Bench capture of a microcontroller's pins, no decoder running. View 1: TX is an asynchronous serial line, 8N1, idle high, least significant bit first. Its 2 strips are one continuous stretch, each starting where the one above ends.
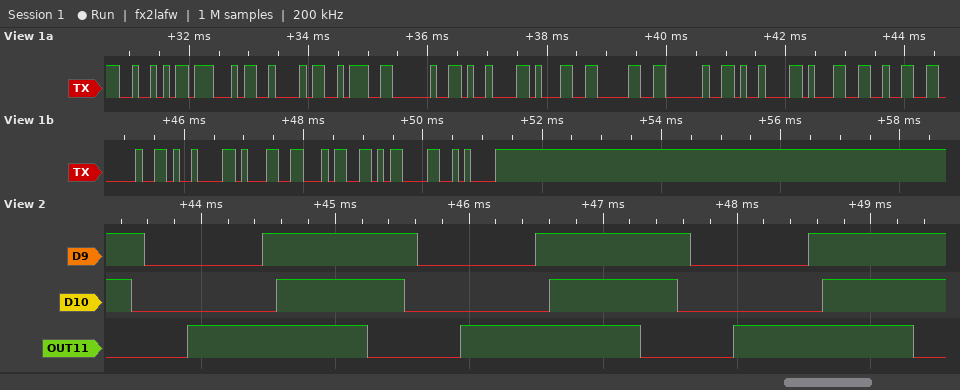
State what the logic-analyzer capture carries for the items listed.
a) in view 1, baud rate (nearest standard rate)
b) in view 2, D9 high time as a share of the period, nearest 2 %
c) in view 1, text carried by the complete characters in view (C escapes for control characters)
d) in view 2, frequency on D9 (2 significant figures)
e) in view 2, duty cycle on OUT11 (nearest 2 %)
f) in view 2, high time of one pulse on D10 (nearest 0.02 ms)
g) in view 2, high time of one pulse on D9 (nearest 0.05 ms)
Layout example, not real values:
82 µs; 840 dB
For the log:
9600 baud; 56 %; "RGB: \t10 \t12 \t14\r\n"; 490 Hz; 66 %; 0.96 ms; 1.15 ms
